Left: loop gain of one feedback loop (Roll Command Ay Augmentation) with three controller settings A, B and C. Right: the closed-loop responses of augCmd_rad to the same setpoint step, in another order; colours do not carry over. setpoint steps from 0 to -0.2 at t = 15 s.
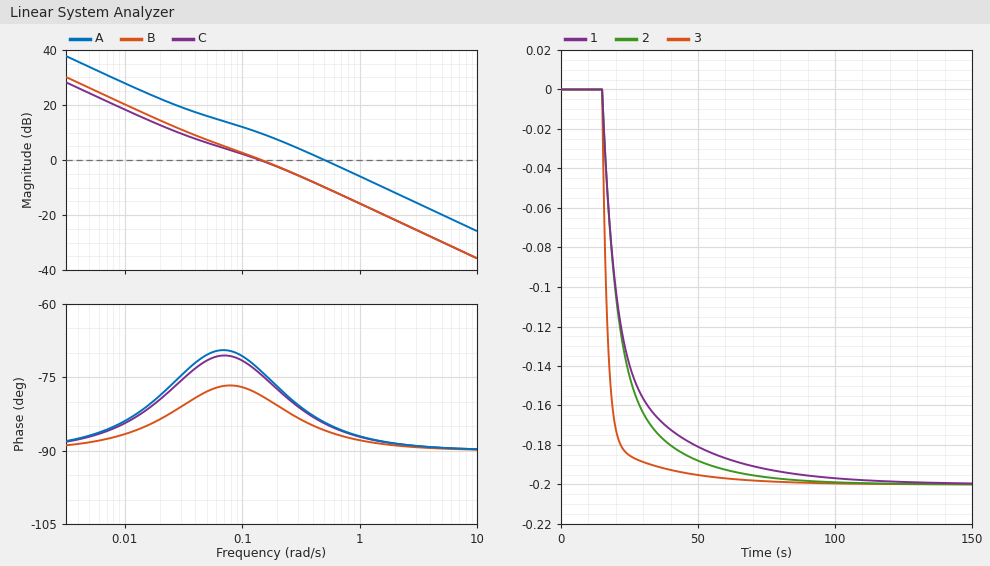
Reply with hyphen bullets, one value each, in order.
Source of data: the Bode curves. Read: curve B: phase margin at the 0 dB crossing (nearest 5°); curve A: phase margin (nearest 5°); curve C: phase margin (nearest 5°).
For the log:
- 100°
- 95°
- 105°
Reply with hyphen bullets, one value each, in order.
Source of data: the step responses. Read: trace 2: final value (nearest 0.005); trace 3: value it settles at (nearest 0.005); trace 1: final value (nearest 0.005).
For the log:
- -0.200
- -0.200
- -0.200
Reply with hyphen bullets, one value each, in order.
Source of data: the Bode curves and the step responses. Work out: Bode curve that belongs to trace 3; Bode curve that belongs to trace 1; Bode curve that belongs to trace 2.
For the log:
- A
- C
- B
